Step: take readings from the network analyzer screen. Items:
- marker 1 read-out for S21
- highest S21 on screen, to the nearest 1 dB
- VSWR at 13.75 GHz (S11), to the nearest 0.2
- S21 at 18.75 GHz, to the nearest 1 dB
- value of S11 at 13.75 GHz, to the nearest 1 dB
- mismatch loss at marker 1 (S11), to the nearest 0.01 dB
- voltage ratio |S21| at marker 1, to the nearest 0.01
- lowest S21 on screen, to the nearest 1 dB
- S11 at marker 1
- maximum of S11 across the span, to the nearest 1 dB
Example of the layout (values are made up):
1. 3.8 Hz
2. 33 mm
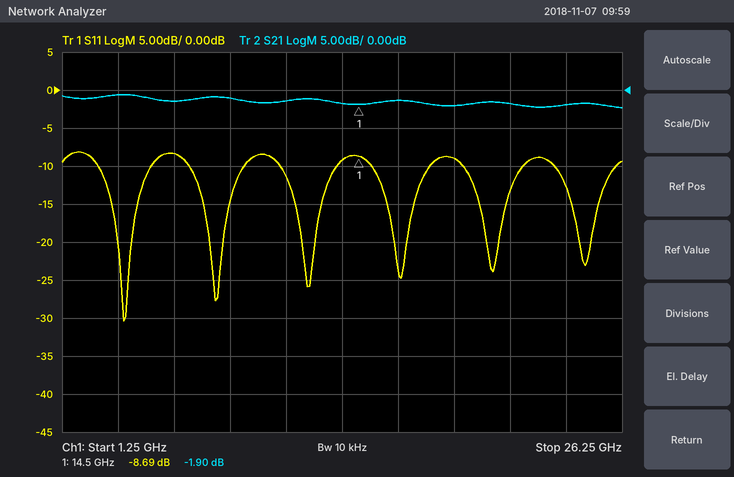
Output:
1. -1.90 dB
2. -1 dB
3. 2.0
4. -2 dB
5. -9 dB
6. 0.63 dB
7. 0.80
8. -2 dB
9. -8.69 dB
10. -8 dB
